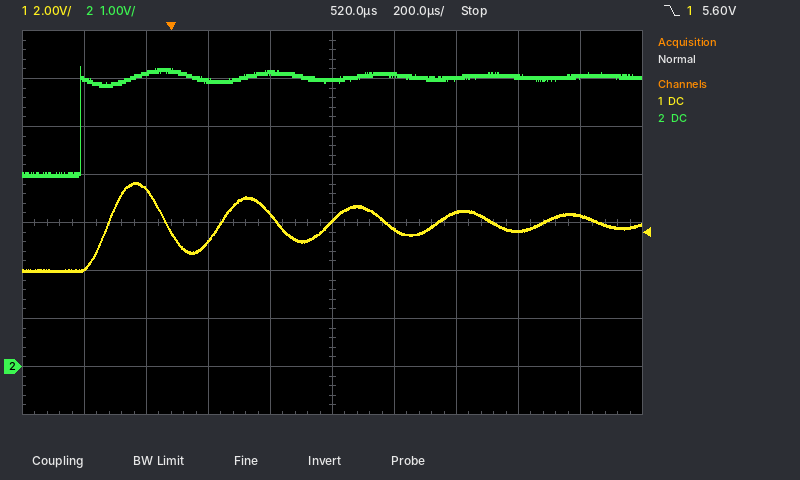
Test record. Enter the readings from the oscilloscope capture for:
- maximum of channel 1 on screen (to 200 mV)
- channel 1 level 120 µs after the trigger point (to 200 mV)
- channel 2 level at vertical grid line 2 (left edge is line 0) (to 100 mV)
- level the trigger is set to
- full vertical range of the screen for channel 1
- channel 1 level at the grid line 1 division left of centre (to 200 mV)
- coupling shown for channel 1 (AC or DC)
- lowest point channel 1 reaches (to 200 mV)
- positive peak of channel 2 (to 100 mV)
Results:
7.6 V
5.2 V
6.1 V
5.60 V
16 V
6.4 V
DC
4.0 V
6.2 V
